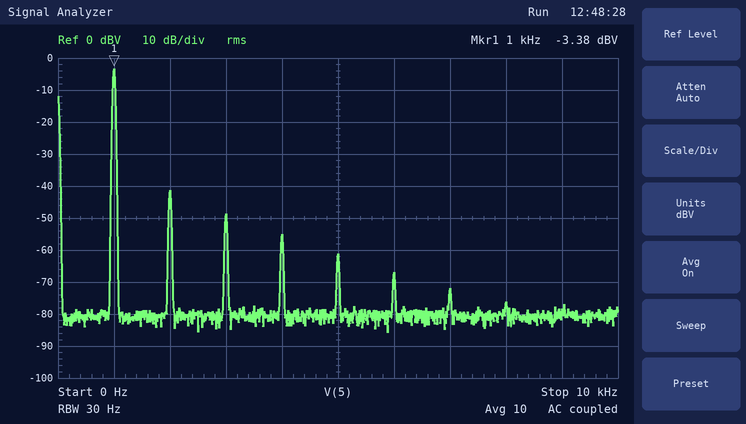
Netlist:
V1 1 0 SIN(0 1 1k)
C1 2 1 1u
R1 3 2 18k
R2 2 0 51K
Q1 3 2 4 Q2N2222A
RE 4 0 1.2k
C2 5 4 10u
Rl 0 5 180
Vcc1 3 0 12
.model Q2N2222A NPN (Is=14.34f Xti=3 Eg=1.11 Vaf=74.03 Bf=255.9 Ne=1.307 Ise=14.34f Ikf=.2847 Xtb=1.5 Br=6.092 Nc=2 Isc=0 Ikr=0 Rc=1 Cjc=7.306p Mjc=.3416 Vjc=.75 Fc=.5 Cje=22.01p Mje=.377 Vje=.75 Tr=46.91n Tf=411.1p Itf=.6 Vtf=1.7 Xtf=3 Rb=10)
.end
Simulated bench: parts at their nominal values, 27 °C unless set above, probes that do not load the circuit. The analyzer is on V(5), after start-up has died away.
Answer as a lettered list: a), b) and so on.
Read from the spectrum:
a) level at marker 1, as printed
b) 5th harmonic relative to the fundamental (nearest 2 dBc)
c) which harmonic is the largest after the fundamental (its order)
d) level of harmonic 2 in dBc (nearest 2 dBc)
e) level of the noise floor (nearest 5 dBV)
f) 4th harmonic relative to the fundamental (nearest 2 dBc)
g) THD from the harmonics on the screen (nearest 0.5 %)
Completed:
a) -3.38 dBV
b) -58 dBc
c) 2
d) -38 dBc
e) -80 dBV
f) -52 dBc
g) 1.5 %
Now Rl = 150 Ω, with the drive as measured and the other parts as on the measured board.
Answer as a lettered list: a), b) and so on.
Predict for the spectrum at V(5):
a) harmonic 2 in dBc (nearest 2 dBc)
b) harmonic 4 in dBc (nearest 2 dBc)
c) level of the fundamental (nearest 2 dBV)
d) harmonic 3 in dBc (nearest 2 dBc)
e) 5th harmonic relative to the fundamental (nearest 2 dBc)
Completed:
a) -30 dBc
b) -38 dBc
c) -4 dBV
d) -34 dBc
e) -42 dBc
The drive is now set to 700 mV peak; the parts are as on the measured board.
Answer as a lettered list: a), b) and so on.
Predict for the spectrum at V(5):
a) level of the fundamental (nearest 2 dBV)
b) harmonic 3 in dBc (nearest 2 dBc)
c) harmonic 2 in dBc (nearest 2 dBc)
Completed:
a) -6 dBV
b) -58 dBc
c) -46 dBc
